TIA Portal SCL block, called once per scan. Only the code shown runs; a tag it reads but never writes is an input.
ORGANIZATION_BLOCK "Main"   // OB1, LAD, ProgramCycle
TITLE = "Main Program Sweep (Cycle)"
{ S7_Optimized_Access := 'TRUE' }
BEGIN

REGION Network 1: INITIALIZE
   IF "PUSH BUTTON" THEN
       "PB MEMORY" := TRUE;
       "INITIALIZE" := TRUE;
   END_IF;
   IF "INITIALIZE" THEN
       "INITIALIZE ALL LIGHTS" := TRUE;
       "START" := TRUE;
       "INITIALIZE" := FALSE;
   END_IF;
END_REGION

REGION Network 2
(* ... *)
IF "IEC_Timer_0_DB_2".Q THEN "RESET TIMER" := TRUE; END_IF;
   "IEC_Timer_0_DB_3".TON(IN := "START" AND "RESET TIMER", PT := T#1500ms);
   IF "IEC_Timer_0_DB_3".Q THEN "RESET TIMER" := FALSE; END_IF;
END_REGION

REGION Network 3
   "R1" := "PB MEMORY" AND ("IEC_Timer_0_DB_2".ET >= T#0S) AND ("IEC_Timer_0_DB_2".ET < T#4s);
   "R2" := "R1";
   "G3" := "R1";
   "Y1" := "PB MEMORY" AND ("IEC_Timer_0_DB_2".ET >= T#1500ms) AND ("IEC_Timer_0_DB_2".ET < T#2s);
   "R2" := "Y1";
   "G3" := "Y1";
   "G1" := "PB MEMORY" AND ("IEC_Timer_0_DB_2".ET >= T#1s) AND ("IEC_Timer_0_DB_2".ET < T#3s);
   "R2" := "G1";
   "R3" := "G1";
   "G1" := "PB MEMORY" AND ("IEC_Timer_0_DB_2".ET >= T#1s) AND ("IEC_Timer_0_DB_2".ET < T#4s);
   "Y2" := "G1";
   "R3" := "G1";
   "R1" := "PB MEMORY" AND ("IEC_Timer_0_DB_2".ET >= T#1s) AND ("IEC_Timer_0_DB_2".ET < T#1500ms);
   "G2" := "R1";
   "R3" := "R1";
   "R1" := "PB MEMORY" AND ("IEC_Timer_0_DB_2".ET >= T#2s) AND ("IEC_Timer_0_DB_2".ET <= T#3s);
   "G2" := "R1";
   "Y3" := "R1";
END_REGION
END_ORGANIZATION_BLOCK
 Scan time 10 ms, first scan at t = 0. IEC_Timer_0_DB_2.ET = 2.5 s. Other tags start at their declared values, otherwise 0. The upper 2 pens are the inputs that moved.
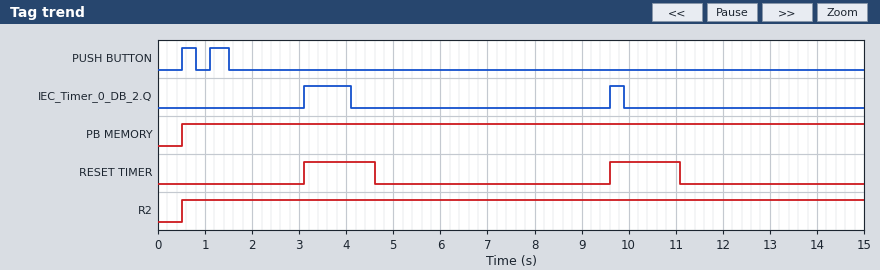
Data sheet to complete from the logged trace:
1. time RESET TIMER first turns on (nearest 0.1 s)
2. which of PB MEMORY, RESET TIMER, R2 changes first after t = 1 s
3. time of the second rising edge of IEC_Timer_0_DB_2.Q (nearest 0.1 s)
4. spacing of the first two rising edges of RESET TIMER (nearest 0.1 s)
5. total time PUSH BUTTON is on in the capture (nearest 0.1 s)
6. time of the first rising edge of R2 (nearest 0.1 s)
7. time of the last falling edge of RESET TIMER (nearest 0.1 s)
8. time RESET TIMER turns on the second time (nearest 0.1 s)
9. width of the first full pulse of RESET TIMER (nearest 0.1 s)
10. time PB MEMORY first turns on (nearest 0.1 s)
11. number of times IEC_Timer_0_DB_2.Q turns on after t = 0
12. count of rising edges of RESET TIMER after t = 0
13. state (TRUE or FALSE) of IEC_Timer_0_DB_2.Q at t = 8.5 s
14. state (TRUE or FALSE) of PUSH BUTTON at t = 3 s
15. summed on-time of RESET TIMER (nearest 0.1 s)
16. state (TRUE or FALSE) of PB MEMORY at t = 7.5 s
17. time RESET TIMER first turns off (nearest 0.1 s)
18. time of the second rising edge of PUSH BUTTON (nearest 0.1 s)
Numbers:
3.1 s
RESET TIMER
9.6 s
6.5 s
0.7 s
0.5 s
11.1 s
9.6 s
1.5 s
0.5 s
2
2
FALSE
FALSE
3.0 s
TRUE
4.6 s
1.1 s
